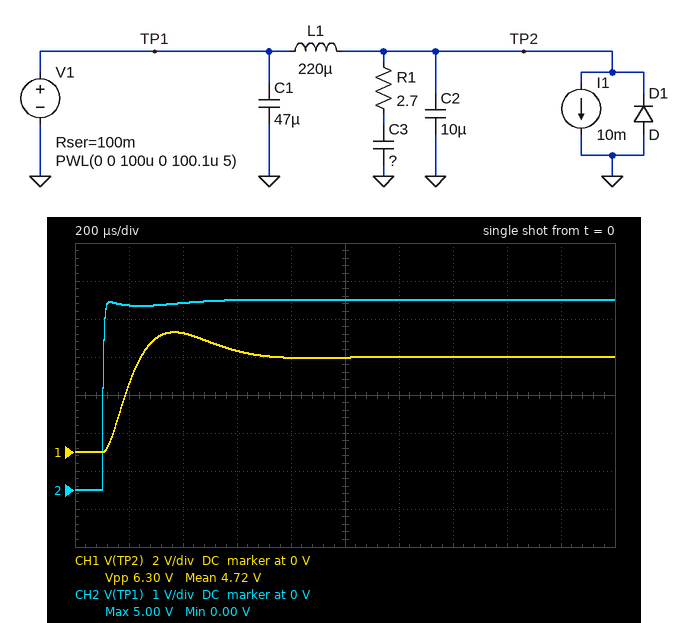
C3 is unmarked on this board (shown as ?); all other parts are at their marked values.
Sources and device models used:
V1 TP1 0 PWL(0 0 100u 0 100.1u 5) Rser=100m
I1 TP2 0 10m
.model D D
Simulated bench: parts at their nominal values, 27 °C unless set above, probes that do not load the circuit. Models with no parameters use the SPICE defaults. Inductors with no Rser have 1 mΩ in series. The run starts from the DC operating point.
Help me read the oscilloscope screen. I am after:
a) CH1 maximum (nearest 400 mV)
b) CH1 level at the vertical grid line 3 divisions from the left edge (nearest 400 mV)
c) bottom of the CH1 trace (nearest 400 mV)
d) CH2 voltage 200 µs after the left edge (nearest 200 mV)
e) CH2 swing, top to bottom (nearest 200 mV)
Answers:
6.4 V
5.2 V
0 V
4.8 V
5.0 V
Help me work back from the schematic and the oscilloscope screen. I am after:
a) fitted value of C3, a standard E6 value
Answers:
68 µF
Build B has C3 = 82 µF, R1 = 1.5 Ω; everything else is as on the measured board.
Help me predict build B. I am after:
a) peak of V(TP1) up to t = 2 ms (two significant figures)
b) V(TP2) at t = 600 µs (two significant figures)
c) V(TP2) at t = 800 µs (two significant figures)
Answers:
5.0 V
6.1 V
4.8 V
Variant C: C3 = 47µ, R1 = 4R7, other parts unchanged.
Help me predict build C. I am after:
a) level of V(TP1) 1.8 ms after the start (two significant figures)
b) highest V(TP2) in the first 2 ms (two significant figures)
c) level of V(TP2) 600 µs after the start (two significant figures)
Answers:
5.0 V
6.6 V
5.1 V
